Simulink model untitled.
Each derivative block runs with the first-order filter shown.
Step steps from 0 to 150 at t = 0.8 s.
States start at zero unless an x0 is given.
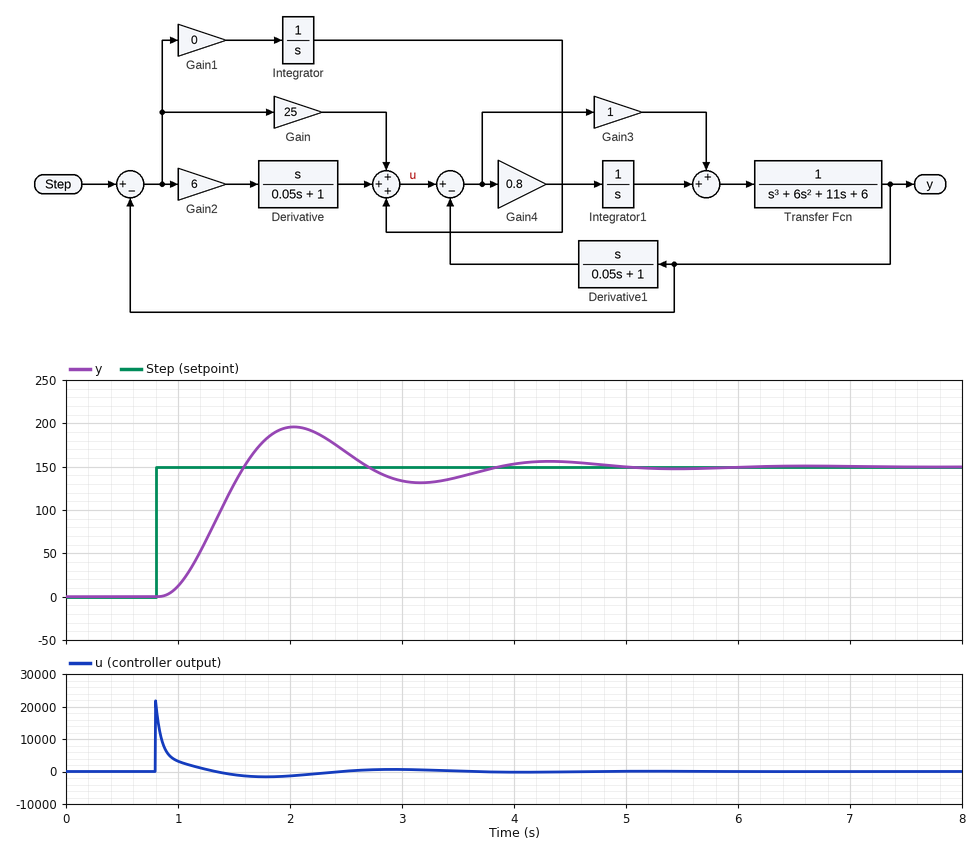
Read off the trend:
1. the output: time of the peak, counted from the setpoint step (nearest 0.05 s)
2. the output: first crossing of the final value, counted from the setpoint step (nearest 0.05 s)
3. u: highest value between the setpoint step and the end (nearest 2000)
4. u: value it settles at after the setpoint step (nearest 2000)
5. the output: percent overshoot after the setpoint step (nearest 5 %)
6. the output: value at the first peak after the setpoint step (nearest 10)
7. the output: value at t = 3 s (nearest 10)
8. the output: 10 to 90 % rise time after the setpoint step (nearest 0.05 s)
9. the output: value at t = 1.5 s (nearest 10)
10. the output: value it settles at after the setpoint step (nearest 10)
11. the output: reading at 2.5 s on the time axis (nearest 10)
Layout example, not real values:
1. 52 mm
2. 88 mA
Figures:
1. 1.25 s
2. 0.80 s
3. 22000
4. 0
5. 30 %
6. 200
7. 130
8. 0.50 s
9. 130
10. 150
11. 170
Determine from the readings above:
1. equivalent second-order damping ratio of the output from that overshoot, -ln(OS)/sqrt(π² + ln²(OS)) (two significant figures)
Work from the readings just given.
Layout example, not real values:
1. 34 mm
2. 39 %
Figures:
1. 0.36
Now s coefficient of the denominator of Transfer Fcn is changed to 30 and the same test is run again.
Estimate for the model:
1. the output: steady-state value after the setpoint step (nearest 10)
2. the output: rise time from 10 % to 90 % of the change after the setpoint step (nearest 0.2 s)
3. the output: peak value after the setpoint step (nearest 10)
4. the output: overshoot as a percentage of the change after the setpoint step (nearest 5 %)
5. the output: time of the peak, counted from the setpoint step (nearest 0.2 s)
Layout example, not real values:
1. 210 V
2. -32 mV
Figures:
1. 150
2. 1.2 s
3. 170
4. 15 %
5. 3.2 s
